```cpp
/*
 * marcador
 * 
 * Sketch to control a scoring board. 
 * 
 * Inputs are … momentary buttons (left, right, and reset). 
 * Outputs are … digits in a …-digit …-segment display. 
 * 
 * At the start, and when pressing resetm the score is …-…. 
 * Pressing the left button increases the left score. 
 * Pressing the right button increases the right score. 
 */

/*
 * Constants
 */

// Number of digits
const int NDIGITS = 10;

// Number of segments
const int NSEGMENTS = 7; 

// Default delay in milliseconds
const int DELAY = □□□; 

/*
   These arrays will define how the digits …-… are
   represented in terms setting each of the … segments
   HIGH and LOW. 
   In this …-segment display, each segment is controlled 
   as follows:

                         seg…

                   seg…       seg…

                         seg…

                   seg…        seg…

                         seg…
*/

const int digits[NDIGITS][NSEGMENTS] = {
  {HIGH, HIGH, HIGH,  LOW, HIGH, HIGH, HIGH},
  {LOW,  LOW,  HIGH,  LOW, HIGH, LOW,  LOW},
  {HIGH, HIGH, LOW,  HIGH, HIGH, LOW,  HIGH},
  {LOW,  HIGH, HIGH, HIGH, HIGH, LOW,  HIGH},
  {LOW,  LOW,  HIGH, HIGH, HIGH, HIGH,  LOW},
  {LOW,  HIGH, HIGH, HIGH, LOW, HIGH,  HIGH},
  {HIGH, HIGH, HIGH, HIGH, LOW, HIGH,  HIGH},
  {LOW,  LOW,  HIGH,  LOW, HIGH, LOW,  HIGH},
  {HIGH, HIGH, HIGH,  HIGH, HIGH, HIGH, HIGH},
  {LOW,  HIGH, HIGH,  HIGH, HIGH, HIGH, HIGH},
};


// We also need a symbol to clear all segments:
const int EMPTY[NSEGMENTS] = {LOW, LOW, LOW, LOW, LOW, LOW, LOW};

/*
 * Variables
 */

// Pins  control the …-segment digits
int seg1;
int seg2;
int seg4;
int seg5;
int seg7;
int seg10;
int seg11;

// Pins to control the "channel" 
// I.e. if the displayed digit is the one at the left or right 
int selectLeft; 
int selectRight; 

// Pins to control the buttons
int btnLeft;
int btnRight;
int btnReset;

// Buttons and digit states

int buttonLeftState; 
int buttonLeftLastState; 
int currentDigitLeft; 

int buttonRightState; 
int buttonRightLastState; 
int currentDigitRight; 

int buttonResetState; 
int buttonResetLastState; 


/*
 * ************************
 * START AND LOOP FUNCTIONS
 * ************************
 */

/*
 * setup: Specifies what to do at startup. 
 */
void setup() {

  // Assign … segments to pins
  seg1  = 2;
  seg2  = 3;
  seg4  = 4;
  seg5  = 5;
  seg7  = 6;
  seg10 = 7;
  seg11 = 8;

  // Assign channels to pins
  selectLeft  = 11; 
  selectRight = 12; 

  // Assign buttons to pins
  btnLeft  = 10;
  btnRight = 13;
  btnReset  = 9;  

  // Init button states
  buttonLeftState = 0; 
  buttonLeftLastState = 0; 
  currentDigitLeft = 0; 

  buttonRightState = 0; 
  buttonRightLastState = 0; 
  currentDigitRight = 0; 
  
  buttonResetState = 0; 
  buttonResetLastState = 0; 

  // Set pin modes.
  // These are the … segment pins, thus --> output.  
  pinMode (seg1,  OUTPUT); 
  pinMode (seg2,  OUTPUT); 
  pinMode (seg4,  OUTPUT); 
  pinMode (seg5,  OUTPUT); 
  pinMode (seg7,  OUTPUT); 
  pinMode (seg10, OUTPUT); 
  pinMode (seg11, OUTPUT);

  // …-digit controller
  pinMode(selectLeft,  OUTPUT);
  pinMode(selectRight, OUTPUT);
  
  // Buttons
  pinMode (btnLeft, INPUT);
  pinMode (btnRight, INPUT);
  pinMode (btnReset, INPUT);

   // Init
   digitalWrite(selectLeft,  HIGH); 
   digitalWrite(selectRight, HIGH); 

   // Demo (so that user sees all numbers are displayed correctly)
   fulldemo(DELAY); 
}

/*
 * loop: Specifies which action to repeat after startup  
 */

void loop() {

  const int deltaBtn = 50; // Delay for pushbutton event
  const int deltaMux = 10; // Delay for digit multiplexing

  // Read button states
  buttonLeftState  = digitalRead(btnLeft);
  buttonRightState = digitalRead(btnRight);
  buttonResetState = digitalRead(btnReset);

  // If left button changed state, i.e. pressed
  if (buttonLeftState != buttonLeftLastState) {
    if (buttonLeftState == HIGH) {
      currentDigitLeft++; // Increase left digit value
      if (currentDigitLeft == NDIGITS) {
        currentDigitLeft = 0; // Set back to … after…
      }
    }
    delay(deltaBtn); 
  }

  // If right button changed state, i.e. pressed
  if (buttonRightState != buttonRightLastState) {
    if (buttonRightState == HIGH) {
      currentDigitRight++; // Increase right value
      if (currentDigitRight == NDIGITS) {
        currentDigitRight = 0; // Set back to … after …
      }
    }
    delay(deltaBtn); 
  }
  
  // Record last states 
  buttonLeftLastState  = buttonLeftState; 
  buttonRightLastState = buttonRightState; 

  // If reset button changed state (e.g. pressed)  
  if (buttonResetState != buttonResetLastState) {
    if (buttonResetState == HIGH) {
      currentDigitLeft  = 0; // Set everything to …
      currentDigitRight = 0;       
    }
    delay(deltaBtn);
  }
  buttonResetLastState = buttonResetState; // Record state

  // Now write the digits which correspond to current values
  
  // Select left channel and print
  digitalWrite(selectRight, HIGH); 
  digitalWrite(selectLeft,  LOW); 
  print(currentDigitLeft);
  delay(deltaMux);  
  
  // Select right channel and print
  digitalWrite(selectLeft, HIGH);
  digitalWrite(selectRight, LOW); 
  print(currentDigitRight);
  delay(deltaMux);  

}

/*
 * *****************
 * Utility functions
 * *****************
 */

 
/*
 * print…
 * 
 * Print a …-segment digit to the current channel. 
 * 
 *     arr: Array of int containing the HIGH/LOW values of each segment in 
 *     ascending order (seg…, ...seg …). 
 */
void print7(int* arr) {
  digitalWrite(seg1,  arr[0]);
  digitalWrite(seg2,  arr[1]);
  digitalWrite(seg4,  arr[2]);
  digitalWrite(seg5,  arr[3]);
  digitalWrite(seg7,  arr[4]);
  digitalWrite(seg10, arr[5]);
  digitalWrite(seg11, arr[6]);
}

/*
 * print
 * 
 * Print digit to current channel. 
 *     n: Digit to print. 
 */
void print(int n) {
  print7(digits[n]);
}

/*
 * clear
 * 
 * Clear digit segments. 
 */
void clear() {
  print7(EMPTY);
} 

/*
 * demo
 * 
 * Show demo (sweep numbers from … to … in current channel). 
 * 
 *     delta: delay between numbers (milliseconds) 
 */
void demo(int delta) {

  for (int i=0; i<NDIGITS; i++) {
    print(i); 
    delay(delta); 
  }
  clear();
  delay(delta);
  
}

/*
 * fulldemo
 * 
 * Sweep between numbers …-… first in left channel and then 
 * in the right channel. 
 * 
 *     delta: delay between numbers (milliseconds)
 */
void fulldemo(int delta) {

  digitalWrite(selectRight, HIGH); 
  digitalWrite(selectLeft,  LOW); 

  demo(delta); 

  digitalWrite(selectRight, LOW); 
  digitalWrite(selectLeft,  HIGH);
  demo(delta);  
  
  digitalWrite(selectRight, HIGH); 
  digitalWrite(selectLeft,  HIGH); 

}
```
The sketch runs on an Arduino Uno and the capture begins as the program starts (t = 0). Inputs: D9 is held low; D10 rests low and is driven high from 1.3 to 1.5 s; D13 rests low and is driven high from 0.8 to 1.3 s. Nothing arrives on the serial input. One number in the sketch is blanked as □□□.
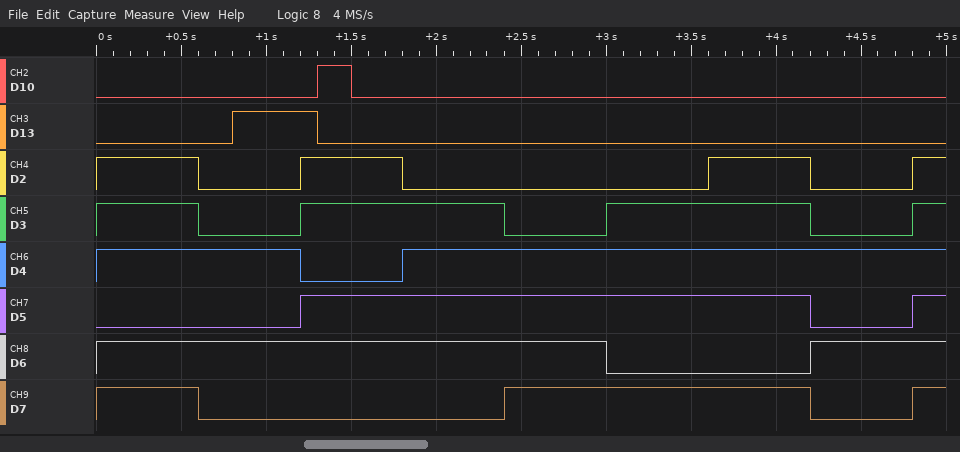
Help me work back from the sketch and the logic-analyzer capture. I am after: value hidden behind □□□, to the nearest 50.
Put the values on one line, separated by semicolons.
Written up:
600
